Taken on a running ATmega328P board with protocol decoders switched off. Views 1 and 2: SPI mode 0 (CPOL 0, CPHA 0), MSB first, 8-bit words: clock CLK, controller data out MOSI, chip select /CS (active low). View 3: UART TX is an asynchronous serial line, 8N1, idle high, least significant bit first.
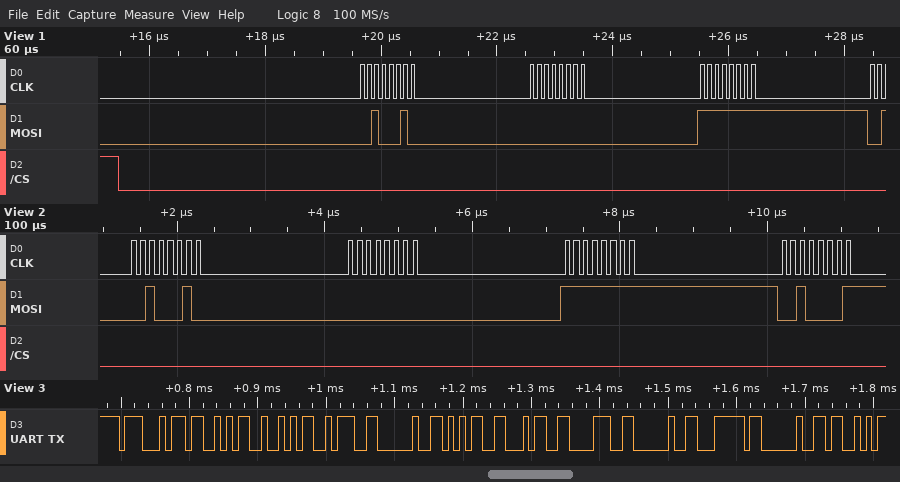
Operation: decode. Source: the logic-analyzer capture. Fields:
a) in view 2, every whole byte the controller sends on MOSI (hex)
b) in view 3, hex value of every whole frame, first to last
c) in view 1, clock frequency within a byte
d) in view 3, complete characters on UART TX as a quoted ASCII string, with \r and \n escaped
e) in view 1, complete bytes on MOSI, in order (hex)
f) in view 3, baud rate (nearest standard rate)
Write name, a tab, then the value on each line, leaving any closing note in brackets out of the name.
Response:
in view 2, every whole byte the controller sends on MOSI	22 00 FF 21
in view 3, hex value of every whole frame, first to last	0x47 0x53 0x52 0x3A 0x20 0x35 0x34 0x38 0x20 0x7C 0x20 0x53
in view 1, clock frequency within a byte	8 MHz
in view 3, complete characters on UART TX as a quoted ASCII string, with \r and \n escaped	"GSR: 548 | S"
in view 1, complete bytes on MOSI, in order	0x22 0x00 0xFF
in view 3, baud rate	115200 baud
